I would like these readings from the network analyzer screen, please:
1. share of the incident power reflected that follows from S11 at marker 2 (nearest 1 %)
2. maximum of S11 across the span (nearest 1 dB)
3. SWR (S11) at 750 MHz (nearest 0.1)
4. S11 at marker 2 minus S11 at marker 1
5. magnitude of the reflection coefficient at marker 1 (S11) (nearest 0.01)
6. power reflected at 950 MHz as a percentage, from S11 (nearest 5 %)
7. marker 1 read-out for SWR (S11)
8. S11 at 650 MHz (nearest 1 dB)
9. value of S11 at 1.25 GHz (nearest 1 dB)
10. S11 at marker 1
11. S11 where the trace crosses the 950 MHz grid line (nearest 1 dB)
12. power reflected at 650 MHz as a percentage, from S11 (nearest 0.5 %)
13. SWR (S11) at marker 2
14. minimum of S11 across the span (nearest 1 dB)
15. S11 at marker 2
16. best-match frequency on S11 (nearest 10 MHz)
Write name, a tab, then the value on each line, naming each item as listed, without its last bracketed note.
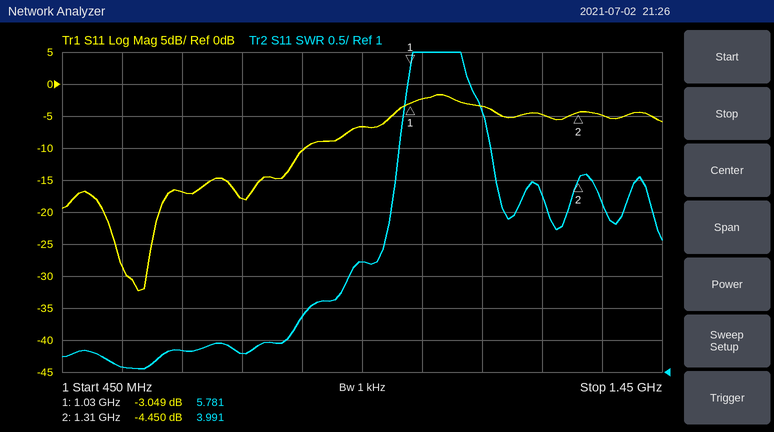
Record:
share of the incident power reflected that follows from S11 at marker 2	36 %
maximum of S11 across the span	-2 dB
SWR (S11) at 750 MHz	1.3
S11 at marker 2 minus S11 at marker 1	-1.401 dB
magnitude of the reflection coefficient at marker 1 (S11)	0.70
power reflected at 950 MHz as a percentage, from S11	20 %
marker 1 read-out for SWR	5.781
S11 at 650 MHz	-17 dB
value of S11 at 1.25 GHz	-5 dB
S11 at marker 1	-3.049 dB
S11 where the trace crosses the 950 MHz grid line	-7 dB
power reflected at 650 MHz as a percentage, from S11	2.0 %
SWR (S11) at marker 2	3.991
minimum of S11 across the span	-32 dB
S11 at marker 2	-4.450 dB
best-match frequency on S11	580 MHz
